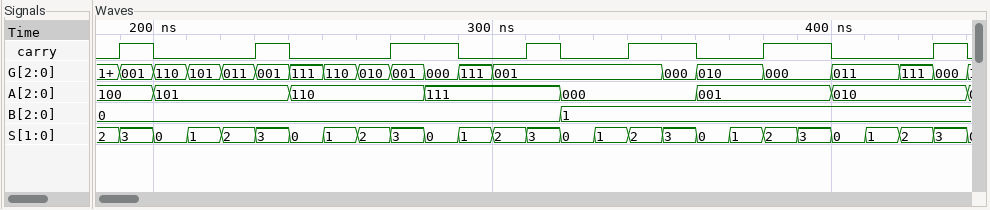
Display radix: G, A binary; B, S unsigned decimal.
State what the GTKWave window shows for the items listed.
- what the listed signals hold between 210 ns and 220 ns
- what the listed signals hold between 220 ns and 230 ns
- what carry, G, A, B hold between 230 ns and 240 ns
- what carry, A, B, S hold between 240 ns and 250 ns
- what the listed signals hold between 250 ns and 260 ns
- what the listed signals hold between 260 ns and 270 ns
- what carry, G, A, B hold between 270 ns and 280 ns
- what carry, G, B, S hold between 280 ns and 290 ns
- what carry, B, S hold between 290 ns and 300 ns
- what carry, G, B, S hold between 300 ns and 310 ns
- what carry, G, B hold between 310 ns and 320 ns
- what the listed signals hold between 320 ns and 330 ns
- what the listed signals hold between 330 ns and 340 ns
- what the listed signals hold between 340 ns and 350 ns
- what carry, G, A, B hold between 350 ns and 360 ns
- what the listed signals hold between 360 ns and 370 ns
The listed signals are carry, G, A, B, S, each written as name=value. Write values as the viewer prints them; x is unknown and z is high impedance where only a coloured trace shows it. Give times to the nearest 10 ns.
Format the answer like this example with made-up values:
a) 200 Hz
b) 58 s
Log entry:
a) carry=0, G=101, A=101, B=0, S=1
b) carry=0, G=011, A=101, B=0, S=2
c) carry=1, G=001, A=101, B=0
d) carry=0, A=110, B=0, S=0
e) carry=0, G=110, A=110, B=0, S=1
f) carry=0, G=010, A=110, B=0, S=2
g) carry=1, G=001, A=110, B=0
h) carry=1, G=000, B=0, S=0
i) carry=0, B=0, S=1
j) carry=0, G=001, B=0, S=2
k) carry=1, G=001, B=0
l) carry=0, G=001, A=000, B=1, S=0
m) carry=0, G=001, A=000, B=1, S=1
n) carry=1, G=001, A=000, B=1, S=2
o) carry=1, G=000, A=000, B=1
p) carry=0, G=010, A=001, B=1, S=0
